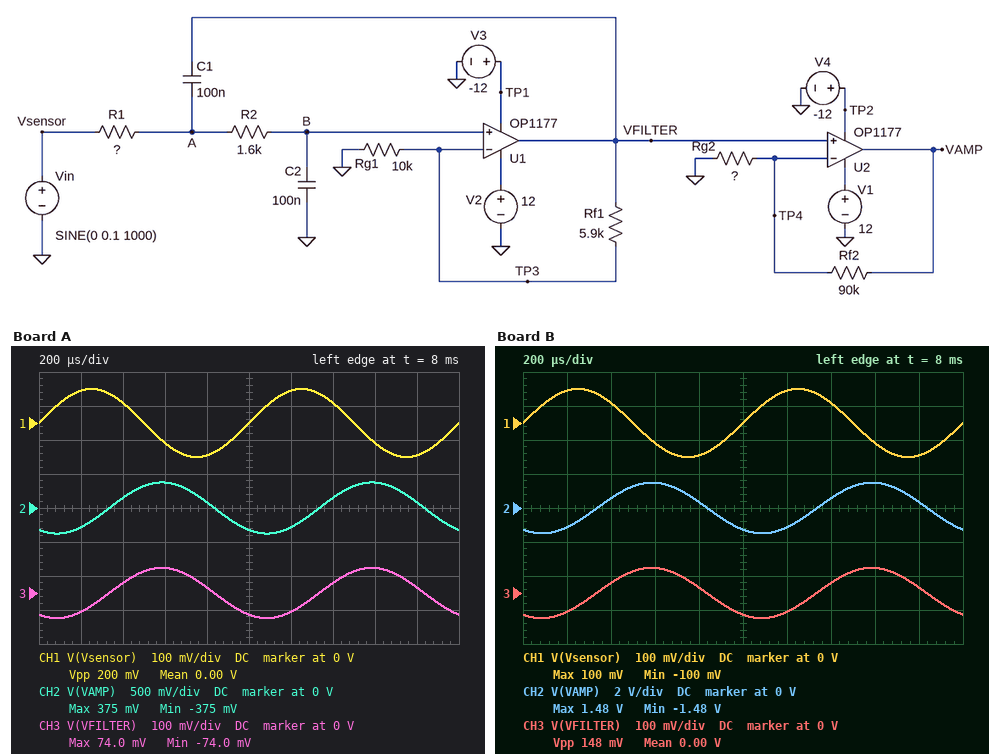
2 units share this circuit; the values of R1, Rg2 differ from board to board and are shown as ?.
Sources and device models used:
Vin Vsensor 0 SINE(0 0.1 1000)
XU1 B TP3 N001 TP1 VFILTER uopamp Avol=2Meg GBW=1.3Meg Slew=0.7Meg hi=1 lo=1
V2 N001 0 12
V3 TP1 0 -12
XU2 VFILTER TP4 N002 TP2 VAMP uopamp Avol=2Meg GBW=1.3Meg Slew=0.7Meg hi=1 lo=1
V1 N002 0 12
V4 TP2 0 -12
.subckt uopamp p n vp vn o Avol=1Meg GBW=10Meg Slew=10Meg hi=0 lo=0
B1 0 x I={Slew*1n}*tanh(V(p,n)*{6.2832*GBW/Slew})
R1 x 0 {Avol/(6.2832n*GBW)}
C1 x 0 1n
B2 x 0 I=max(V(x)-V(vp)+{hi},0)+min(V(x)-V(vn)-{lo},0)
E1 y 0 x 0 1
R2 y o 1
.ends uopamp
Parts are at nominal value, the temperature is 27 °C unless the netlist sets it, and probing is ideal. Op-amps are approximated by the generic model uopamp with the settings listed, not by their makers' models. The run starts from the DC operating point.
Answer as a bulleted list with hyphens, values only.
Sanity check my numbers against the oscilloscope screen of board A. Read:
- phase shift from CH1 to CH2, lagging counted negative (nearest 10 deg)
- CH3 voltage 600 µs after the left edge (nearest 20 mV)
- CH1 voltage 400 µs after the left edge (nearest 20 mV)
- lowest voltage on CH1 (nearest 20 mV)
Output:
- -120 deg
- 80 mV
- 60 mV
- -100 mV
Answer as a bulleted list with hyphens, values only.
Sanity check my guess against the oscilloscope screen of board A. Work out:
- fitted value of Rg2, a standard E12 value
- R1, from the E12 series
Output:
- 22 kΩ
- 3.3 kΩ
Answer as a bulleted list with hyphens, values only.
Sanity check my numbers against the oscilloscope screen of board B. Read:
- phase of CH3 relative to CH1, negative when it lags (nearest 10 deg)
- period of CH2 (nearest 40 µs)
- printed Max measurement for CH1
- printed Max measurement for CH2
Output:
- -120 deg
- 1.00 ms
- 100 mV
- 1.48 V
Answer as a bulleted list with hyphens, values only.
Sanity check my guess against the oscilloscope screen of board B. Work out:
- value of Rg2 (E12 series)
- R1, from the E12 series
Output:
- 4.7 kΩ
- 3.3 kΩ
